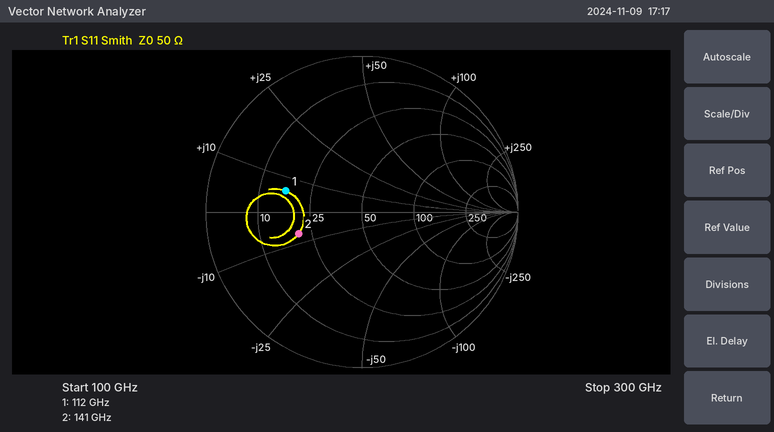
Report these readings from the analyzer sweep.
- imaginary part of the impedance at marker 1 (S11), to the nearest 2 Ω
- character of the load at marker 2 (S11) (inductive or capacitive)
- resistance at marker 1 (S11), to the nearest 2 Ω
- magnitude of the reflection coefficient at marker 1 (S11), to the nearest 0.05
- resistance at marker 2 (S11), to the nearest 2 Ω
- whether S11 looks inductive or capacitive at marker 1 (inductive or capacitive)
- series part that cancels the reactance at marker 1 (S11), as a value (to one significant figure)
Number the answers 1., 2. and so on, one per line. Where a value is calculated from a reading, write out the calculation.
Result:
1. +6 Ω
2. capacitive
3. 16 Ω
4. 0.50
5. 20 Ω
6. inductive
7. C = 1/(2π × 112 GHz × 6 Ω) ≈ 237 fF, so 200 fF to one significant figure
